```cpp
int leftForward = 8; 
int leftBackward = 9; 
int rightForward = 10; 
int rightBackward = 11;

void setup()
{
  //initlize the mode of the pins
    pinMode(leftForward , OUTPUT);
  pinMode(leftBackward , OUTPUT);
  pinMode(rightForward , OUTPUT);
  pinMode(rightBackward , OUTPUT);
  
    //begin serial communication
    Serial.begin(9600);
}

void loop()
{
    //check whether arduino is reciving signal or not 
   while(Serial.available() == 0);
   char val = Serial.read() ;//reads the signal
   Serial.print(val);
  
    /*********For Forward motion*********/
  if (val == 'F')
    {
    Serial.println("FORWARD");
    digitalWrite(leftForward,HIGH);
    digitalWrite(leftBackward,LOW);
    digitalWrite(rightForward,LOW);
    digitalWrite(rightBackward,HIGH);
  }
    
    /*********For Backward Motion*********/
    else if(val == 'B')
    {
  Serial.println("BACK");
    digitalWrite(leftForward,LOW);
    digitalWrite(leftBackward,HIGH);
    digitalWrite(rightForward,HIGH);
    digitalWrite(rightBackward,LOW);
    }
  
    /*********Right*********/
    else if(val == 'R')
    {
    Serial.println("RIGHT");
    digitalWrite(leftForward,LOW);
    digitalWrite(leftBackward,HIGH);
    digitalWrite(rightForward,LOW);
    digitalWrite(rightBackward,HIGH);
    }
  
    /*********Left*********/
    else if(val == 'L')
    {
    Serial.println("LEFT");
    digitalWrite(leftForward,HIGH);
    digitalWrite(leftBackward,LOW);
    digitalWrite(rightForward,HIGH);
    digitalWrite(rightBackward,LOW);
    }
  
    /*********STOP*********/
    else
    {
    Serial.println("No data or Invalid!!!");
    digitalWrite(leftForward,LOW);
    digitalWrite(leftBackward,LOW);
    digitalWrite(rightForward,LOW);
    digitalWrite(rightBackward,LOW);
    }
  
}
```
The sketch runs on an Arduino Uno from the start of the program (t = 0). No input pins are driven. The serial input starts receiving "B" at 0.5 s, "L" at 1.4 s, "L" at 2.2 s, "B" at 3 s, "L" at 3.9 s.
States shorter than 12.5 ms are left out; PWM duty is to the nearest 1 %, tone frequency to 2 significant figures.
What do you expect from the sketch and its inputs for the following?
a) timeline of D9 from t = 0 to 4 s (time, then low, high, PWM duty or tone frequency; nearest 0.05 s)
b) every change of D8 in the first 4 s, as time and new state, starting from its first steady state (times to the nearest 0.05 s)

0 s low; 0.5 s high; 1.4 s low; 3 s high; 3.9 s low
0 s low; 1.4 s high; 3 s low; 3.9 s high
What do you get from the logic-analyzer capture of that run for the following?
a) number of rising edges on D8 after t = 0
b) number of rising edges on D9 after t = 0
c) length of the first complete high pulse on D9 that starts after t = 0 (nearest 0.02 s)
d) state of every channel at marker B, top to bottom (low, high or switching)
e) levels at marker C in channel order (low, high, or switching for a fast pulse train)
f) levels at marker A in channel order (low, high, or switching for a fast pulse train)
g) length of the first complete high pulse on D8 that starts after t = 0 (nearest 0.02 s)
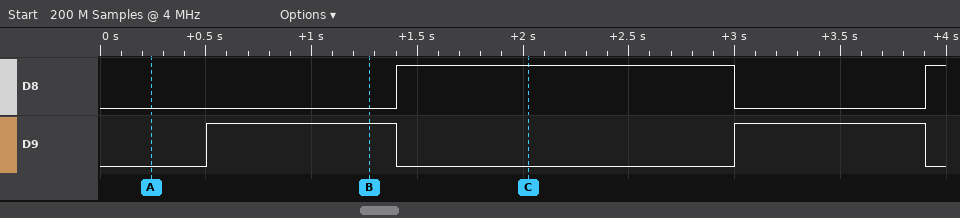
2
2
0.90 s
D8 low, D9 high
D8 high, D9 low
D8 low, D9 low
1.60 s
